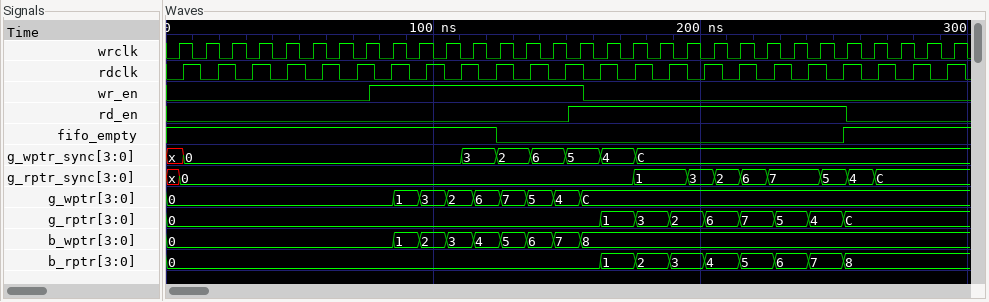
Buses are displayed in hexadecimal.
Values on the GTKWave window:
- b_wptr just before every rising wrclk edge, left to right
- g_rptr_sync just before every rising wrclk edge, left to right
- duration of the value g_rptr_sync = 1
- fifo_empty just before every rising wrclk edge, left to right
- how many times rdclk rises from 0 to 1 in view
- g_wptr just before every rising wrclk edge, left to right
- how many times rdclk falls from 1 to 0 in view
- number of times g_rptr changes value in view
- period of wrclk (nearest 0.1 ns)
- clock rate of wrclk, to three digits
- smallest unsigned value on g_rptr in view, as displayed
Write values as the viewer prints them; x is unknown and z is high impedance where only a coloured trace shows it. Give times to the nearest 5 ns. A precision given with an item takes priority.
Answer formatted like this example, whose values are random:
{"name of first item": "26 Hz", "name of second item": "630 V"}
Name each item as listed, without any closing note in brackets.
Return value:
{"b_wptr just before every rising wrclk edge, left to right": "0, 0, 0, 0, 0, 0, 0, 0, 0, 1, 2, 3, 4, 5, 6, 7, 8, 8, 8, 8, 8, 8, 8, 8, 8, 8, 8, 8, 8, 8", "g_rptr_sync just before every rising wrclk edge, left to right": "x, 0, 0, 0, 0, 0, 0, 0, 0, 0, 0, 0, 0, 0, 0, 0, 0, 0, 1, 1, 3, 2, 6, 7, 7, 5, 4, C, C, C", "duration of the value g_rptr_sync = 1": "20 ns", "fifo_empty just before every rising wrclk edge, left to right": "1 1 1 1 1 1 1 1 1 1 1 1 0 0 0 0 0 0 0 0 0 0 0 0 0 1 1 1 1 1", "how many times rdclk rises from 0 to 1 in view": "23", "g_wptr just before every rising wrclk edge, left to right": "0, 0, 0, 0, 0, 0, 0, 0, 0, 1, 3, 2, 6, 7, 5, 4, C, C, C, C, C, C, C, C, C, C, C, C, C, C", "how many times rdclk falls from 1 to 0 in view": "23", "number of times g_rptr changes value in view": "8", "period of wrclk": "10 ns", "clock rate of wrclk, to three digits": "100 MHz", "smallest unsigned value on g_rptr in view, as displayed": "0"}
